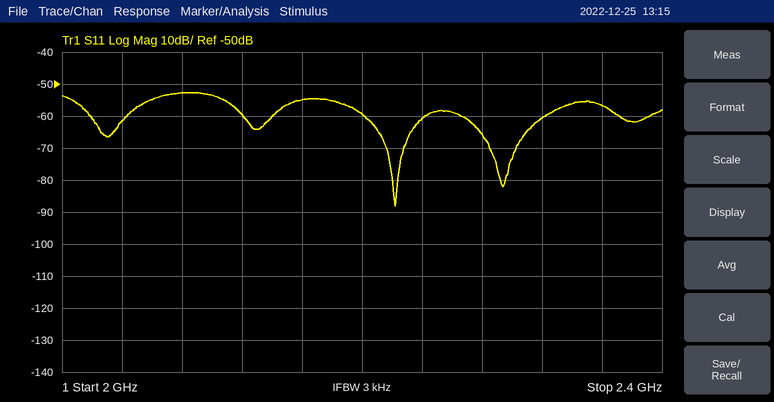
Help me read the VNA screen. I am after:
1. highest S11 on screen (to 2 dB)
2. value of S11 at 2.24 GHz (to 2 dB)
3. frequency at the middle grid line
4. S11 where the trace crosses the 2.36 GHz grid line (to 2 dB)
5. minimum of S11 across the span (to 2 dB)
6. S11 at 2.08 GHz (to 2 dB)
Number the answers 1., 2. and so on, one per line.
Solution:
1. -52 dB
2. -60 dB
3. 2.2 GHz
4. -56 dB
5. -88 dB
6. -52 dB
